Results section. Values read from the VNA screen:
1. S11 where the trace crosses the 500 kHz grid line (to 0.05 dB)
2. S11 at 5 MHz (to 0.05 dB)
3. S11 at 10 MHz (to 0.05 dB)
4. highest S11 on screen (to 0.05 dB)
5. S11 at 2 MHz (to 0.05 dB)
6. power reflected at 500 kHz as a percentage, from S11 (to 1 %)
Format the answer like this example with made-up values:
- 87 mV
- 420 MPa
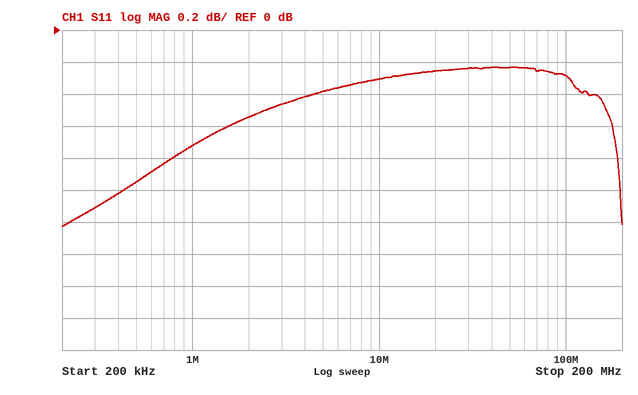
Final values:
- -0.95 dB
- -0.40 dB
- -0.30 dB
- -0.25 dB
- -0.55 dB
- 80 %
